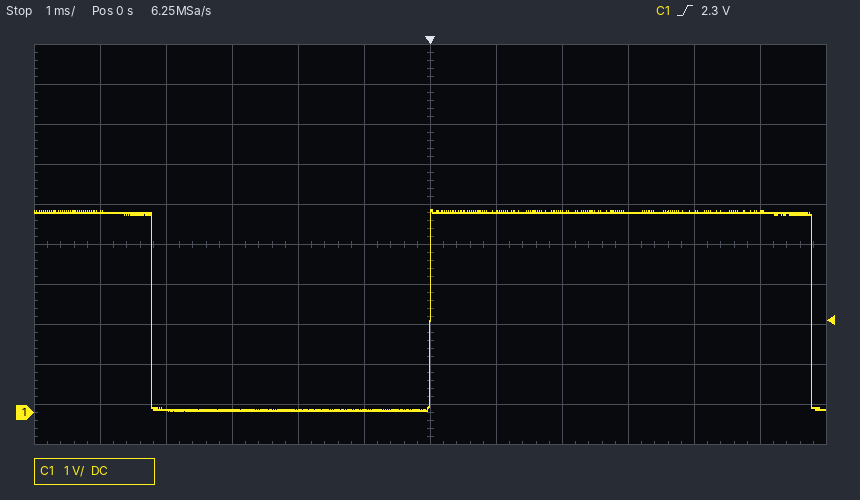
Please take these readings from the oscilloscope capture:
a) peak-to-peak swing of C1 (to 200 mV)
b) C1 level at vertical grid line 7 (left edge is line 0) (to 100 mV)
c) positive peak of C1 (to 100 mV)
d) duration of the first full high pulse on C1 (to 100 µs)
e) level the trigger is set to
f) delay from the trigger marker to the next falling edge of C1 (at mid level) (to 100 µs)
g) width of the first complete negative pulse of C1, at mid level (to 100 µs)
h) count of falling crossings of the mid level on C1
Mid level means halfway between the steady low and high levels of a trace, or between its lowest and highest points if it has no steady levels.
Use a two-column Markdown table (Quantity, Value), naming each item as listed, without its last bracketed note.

| Quantity | Value |
|---|---|
| peak-to-peak swing of C1 | 5.0 V |
| C1 level at vertical grid line 7 (left edge is line 0) | 5.0 V |
| positive peak of C1 | 5.1 V |
| duration of the first full high pulse on C1 | 5.8 ms |
| level the trigger is set to | 2.3 V |
| delay from the trigger marker to the next falling edge of C1 (at mid level) | 5.8 ms |
| width of the first complete negative pulse of C1, at mid level | 4.2 ms |
| count of falling crossings of the mid level on C1 | 2 |
